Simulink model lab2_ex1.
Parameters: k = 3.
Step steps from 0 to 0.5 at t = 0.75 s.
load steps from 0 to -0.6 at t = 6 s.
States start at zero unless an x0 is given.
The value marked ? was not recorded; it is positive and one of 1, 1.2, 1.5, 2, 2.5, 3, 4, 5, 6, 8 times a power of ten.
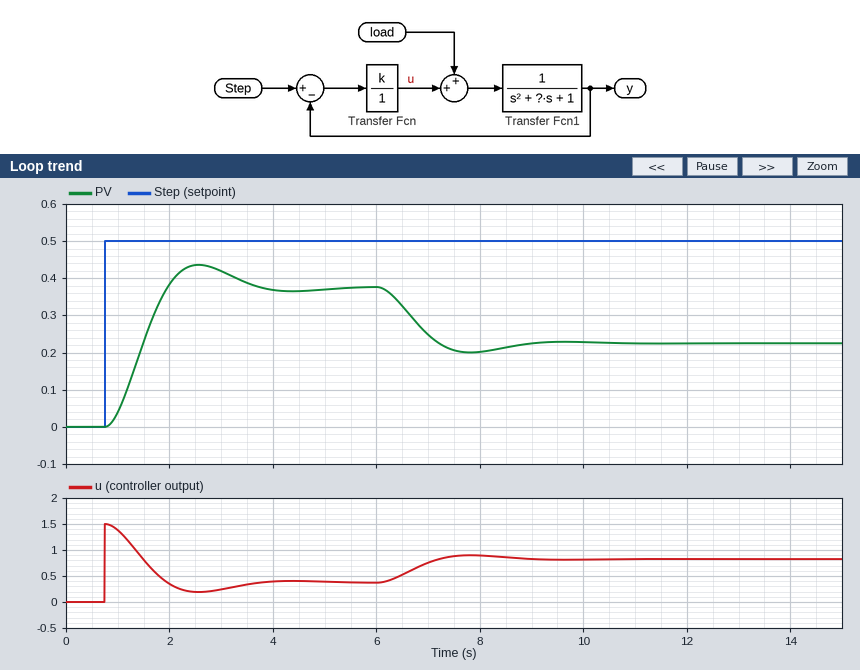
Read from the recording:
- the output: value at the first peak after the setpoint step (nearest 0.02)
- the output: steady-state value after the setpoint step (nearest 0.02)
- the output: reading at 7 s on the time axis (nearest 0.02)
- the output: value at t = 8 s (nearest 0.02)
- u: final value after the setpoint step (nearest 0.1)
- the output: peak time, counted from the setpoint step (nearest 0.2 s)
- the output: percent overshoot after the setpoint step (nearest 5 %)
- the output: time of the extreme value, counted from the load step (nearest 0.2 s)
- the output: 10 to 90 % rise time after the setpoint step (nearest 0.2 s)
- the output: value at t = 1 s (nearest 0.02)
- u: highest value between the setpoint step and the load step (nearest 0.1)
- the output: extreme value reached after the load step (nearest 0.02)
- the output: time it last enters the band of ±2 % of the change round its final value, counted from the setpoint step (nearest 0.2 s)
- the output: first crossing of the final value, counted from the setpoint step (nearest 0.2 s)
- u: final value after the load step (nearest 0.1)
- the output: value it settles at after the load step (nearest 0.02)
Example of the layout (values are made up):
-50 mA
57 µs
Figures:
0.44
0.38
0.24
0.20
0.4
1.8 s
15 %
1.8 s
0.8 s
0.04
1.5
0.20
4.0 s
1.2 s
0.8
0.22
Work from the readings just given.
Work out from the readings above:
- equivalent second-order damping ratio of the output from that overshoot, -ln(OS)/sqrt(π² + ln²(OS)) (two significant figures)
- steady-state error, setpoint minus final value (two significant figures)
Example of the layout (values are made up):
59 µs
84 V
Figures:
0.52
0.12
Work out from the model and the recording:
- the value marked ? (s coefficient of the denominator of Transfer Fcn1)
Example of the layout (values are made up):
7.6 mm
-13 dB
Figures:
2
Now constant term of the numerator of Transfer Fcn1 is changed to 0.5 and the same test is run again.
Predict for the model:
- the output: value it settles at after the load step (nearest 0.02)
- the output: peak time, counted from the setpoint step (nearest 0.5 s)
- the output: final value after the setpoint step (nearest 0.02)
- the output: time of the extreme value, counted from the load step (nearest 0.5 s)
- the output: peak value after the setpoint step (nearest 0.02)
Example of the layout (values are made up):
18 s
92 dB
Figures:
0.18
2.5 s
0.30
2.5 s
0.32
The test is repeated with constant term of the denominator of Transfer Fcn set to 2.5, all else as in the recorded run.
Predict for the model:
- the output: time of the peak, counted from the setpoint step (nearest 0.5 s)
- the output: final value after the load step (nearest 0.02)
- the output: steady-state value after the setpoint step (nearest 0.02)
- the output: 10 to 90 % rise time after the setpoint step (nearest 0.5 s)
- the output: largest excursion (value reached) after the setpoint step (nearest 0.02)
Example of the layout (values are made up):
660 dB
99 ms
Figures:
3.0 s
0.00
0.28
1.5 s
0.28
